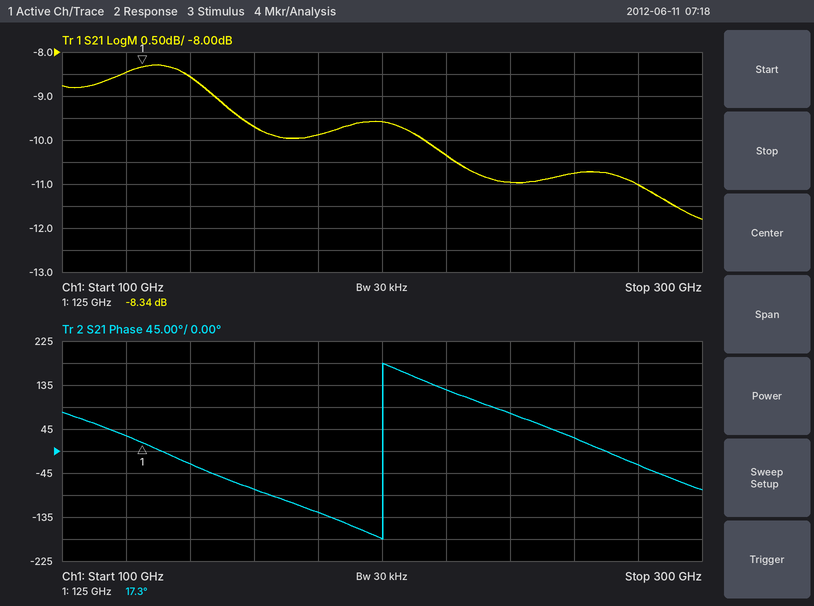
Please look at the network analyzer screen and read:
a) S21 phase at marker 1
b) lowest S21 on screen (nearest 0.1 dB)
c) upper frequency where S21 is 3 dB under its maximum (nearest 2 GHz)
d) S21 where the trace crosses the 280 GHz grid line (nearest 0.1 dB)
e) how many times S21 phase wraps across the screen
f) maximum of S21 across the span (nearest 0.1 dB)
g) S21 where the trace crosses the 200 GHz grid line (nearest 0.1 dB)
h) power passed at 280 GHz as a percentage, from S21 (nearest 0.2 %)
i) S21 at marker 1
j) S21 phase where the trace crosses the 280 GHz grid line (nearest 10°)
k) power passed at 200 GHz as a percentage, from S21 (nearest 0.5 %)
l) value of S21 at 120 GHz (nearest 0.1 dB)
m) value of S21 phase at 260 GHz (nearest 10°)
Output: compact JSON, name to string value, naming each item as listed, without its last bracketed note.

{"S21 phase at marker 1": "17.3°", "lowest S21 on screen": "-11.8 dB", "upper frequency where S21 is 3 dB under its maximum": "286 GHz", "S21 where the trace crosses the 280 GHz grid line": "-11.0 dB", "how many times S21 phase wraps across the screen": "1", "maximum of S21 across the span": "-8.3 dB", "S21 where the trace crosses the 200 GHz grid line": "-9.6 dB", "power passed at 280 GHz as a percentage, from S21": "8.0 %", "S21 at marker 1": "-8.34 dB", "S21 phase where the trace crosses the 280 GHz grid line": "-30°", "power passed at 200 GHz as a percentage, from S21": "11.0 %", "value of S21 at 120 GHz": "-8.5 dB", "value of S21 phase at 260 GHz": "30°"}
